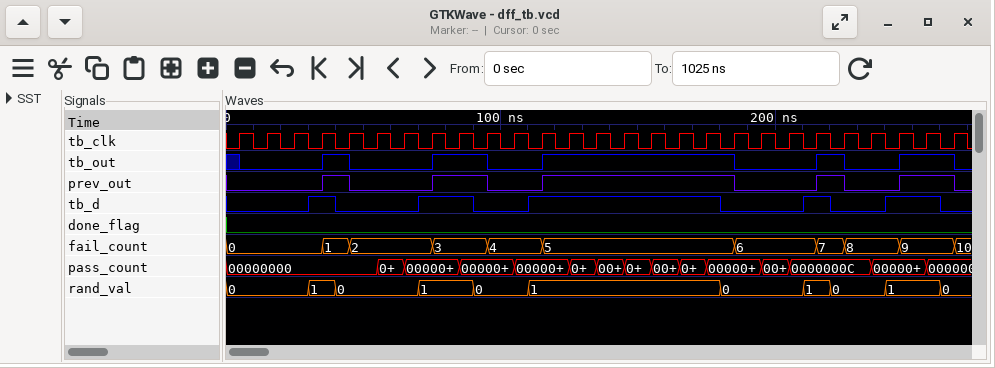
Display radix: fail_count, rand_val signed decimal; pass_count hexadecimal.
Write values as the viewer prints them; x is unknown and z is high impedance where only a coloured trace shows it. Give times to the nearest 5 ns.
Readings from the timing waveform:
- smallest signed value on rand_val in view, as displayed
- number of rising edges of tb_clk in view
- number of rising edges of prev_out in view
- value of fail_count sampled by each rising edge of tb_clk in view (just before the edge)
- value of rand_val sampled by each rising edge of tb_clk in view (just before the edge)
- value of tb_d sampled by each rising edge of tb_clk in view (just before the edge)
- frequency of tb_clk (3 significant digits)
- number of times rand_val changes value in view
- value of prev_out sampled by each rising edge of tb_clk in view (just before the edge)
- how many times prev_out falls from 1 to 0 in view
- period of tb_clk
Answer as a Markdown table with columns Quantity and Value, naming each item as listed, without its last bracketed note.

| Quantity | Value |
|---|---|
| smallest signed value on rand_val in view, as displayed | 0 |
| number of rising edges of tb_clk in view | 27 |
| number of rising edges of prev_out in view | 5 |
| value of fail_count sampled by each rising edge of tb_clk in view | 0, 0, 0, 0, 1, 2, 2, 2, 3, 3, 4, 4, 5, 5, 5, 5, 5, 5, 5, 6, 6, 6, 7, 8, 8, 9, 9 |
| value of rand_val sampled by each rising edge of tb_clk in view | 0, 0, 0, 1, 0, 0, 0, 1, 1, 0, 0, 1, 1, 1, 1, 1, 1, 1, 0, 0, 0, 1, 0, 0, 1, 1, 0 |
| value of tb_d sampled by each rising edge of tb_clk in view | 0 0 0 1 0 0 0 1 1 0 0 1 1 1 1 1 1 1 0 0 0 1 0 0 1 1 0 |
| frequency of tb_clk | 100 MHz |
| number of times rand_val changes value in view | 10 |
| value of prev_out sampled by each rising edge of tb_clk in view | 0 0 0 0 1 0 0 0 1 1 0 0 1 1 1 1 1 1 1 0 0 0 1 0 0 1 1 |
| how many times prev_out falls from 1 to 0 in view | 5 |
| period of tb_clk | 10 ns |
